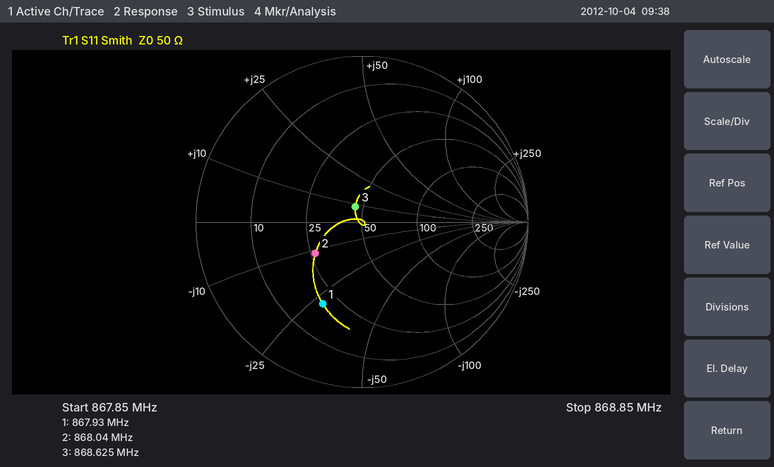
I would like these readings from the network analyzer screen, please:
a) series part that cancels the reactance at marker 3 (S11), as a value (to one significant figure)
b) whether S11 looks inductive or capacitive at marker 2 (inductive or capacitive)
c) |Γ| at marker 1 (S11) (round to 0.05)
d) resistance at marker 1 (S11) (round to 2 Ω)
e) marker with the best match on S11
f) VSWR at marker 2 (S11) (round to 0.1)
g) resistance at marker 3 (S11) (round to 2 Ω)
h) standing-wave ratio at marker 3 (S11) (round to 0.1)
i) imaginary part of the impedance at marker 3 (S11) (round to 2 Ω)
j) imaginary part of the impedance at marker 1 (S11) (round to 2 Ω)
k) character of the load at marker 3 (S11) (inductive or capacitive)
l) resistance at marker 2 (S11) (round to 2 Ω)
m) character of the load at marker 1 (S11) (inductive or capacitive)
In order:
20 pF
capacitive
0.55
20 Ω
marker 3
2.0
46 Ω
1.2
+8 Ω
-28 Ω
inductive
26 Ω
capacitive
